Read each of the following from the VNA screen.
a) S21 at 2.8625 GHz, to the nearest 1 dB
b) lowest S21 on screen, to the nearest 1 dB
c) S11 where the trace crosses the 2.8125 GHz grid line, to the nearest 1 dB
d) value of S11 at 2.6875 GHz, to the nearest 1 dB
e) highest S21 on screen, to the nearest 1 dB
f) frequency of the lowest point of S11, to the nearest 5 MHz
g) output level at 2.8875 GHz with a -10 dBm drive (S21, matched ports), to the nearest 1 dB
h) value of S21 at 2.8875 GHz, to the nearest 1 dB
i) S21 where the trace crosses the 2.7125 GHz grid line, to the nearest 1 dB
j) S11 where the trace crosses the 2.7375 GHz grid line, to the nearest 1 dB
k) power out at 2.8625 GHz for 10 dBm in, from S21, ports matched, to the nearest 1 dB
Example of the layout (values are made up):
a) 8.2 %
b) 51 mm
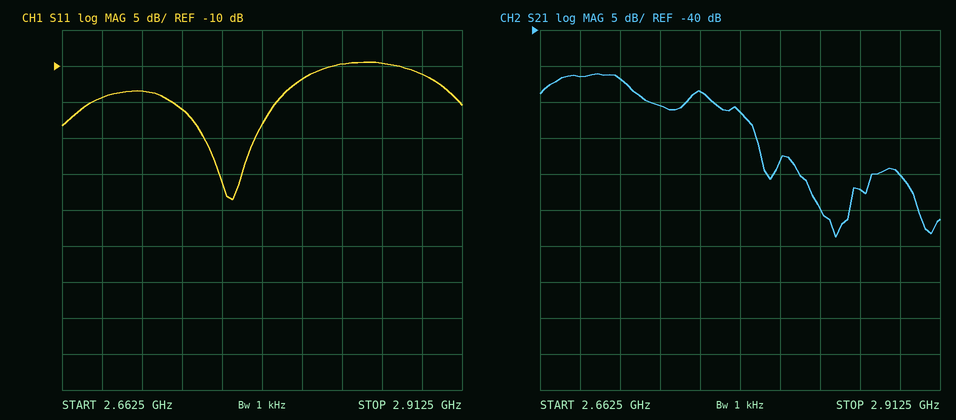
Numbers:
a) -62 dB
b) -69 dB
c) -12 dB
d) -14 dB
e) -46 dB
f) 2.770 GHz
g) -70 dBm
h) -60 dB
i) -47 dB
j) -16 dB
k) -52 dBm
